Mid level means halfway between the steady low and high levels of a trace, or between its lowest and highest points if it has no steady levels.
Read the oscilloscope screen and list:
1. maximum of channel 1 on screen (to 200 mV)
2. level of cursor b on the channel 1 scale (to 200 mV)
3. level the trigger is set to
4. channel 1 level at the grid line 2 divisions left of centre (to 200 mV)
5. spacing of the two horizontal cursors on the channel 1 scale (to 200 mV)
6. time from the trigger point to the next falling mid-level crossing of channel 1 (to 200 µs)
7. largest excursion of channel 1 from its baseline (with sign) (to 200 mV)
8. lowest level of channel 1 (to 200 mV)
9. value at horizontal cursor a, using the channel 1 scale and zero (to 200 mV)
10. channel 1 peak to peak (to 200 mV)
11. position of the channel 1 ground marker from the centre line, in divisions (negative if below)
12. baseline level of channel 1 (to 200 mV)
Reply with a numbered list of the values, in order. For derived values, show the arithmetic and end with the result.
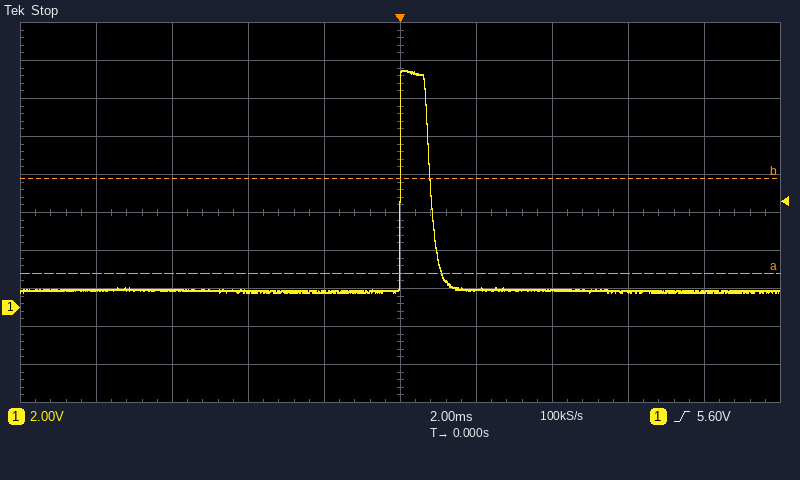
1. 12.4 V
2. 6.8 V
3. 5.60 V
4. 800 mV
5. 5.0 V
6. 800 µs
7. 12.4 V − (800 mV) = +11.6 V
8. 800 mV
9. 1.8 V
10. 12.4 V − (800 mV) = 11.6 V
11. -2.5 div
12. 800 mV
